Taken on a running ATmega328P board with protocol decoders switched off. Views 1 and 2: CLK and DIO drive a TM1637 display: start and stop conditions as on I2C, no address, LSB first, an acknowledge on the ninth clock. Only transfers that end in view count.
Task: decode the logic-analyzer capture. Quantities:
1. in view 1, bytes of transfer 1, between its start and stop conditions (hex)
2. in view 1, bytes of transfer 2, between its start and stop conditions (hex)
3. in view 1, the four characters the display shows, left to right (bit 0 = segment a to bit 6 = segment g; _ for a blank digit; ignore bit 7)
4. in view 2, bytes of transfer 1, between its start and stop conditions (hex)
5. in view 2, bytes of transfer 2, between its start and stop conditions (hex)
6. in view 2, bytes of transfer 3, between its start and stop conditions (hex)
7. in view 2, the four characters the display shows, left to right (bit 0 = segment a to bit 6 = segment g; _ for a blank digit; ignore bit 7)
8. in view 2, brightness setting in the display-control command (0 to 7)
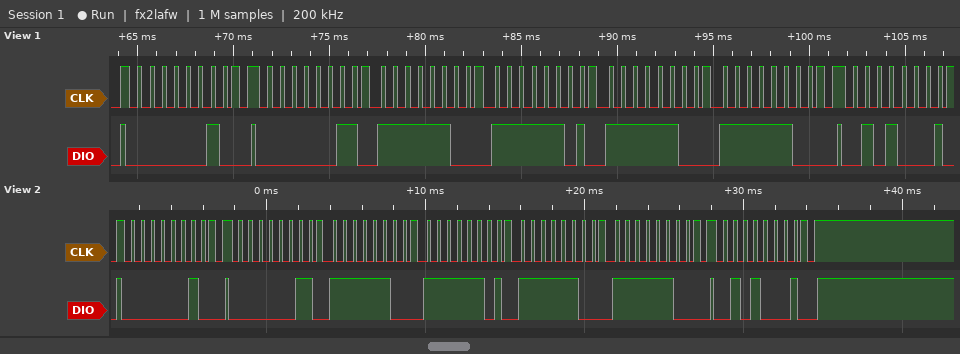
40
C0 3F BF 3F 3F
0000
40
C0 3F BF 3F 3F
8A
0000
2
